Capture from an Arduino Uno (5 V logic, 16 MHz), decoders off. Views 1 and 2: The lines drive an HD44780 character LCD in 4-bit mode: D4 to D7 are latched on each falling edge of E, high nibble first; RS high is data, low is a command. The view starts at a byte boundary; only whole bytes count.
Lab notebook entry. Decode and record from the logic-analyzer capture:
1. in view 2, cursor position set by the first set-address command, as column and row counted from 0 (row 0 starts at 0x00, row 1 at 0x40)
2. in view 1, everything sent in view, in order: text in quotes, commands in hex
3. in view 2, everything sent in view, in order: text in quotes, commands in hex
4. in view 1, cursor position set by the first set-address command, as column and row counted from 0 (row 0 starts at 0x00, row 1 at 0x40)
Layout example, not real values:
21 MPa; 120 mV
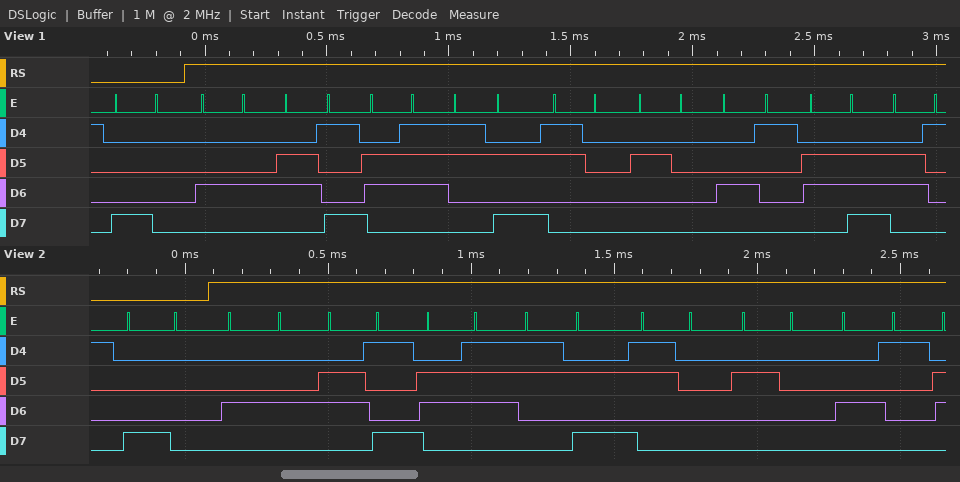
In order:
column 0, row 0; 0x80 "Dig:0 Ana"; 0x80 "Dig:0 A"; column 0, row 0
